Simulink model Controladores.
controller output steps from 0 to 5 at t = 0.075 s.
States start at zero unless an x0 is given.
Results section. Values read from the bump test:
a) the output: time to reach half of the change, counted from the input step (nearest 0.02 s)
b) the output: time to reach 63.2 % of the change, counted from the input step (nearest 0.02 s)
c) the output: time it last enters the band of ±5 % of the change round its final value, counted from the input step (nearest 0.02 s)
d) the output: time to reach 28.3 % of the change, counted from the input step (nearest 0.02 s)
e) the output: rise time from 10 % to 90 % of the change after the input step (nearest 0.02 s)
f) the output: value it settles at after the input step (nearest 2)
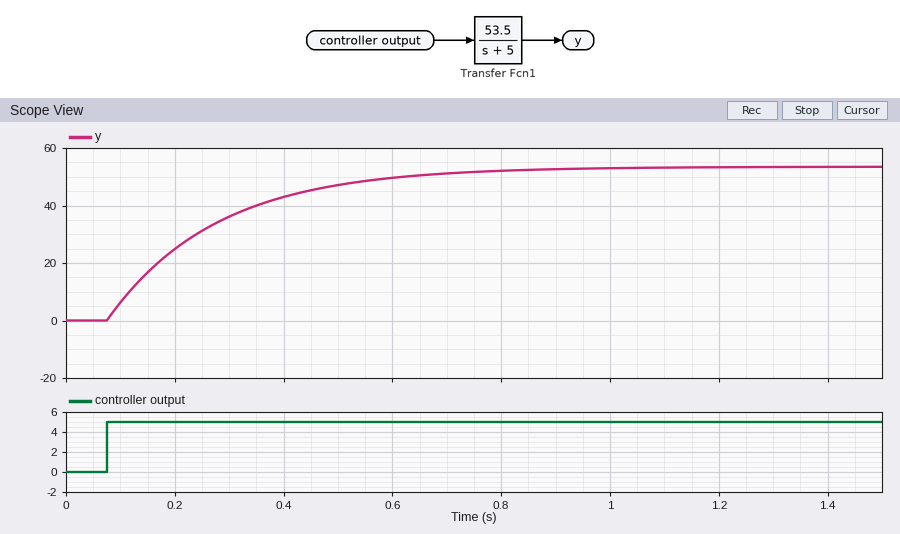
0.14 s
0.20 s
0.60 s
0.06 s
0.44 s
54
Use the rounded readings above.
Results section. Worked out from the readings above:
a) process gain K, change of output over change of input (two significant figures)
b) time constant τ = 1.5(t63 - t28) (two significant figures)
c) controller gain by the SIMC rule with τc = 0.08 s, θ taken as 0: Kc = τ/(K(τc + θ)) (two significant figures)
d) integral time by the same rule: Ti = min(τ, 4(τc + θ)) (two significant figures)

11
0.21 s
0.24
0.21 s
